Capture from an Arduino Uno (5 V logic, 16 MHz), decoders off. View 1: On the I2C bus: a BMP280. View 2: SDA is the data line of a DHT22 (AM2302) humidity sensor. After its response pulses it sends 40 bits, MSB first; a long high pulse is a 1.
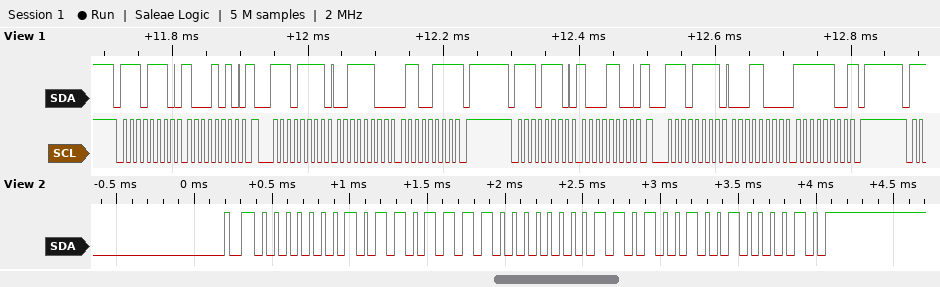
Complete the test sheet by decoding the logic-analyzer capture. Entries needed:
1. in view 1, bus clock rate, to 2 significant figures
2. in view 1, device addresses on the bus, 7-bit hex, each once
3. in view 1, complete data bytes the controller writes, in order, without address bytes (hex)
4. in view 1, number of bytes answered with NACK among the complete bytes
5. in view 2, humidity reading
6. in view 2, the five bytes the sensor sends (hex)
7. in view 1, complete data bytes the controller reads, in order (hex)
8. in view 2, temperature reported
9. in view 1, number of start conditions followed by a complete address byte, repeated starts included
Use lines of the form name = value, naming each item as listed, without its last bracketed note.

in view 1, bus clock rate, to 2 significant figures = 100 kHz
in view 1, device addresses on the bus, 7-bit hex, each once = 0x77
in view 1, complete data bytes the controller writes, in order, without address bytes = 8A 8C
in view 1, number of bytes answered with NACK among the complete bytes = 2
in view 2, humidity reading = 36.7 %
in view 2, the five bytes the sensor sends = 01 6F 00 D2 42
in view 1, complete data bytes the controller reads, in order = 3C 67 18 FC
in view 2, temperature reported = 21.0 °C
in view 1, number of start conditions followed by a complete address byte, repeated starts included = 4
